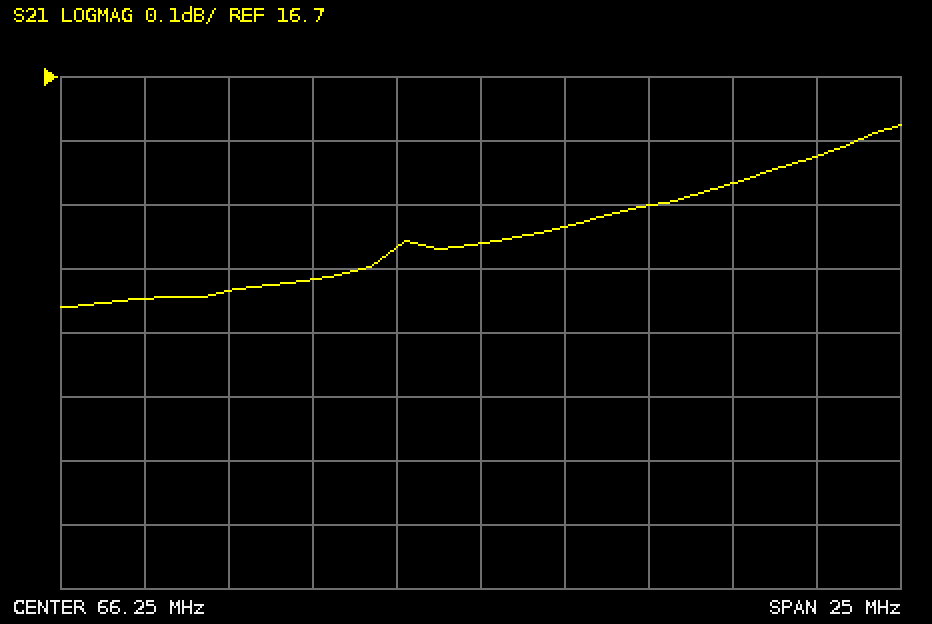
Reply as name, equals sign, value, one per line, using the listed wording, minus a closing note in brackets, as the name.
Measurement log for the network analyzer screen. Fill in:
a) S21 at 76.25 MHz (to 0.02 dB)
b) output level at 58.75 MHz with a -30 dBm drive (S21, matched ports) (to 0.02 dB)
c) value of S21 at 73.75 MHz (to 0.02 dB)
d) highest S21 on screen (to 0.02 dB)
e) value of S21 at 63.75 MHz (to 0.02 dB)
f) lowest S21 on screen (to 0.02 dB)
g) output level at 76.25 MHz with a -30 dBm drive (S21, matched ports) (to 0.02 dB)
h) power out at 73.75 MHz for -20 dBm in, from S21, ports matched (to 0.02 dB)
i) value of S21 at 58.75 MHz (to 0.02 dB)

S21 at 76.25 MHz = 16.58 dB
output level at 58.75 MHz with a -30 dBm drive (S21, matched ports) = -13.64 dBm
value of S21 at 73.75 MHz = 16.54 dB
highest S21 on screen = 16.62 dB
value of S21 at 63.75 MHz = 16.44 dB
lowest S21 on screen = 16.34 dB
output level at 76.25 MHz with a -30 dBm drive (S21, matched ports) = -13.42 dBm
power out at 73.75 MHz for -20 dBm in, from S21, ports matched = -3.46 dBm
value of S21 at 58.75 MHz = 16.36 dB
